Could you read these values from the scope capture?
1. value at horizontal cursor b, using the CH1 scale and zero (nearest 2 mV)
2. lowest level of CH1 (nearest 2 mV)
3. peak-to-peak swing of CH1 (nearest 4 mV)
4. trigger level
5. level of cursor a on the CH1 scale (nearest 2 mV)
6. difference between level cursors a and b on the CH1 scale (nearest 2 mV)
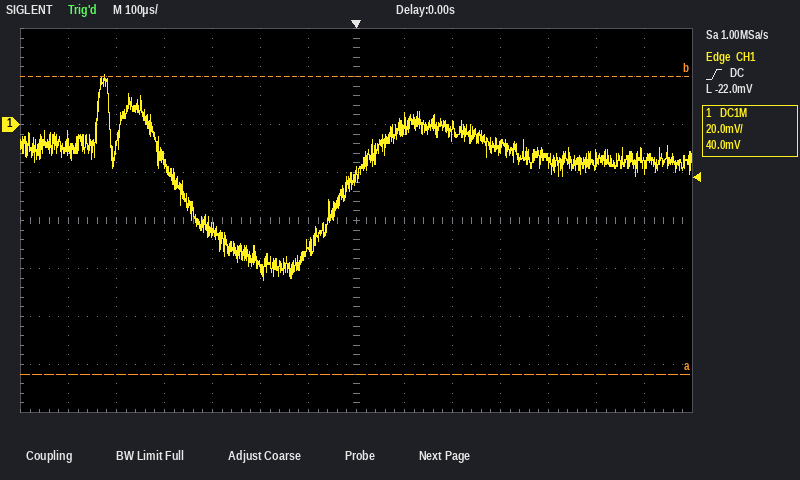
20 mV
-64 mV
84 mV
-22.0 mV
-104 mV
124 mV
